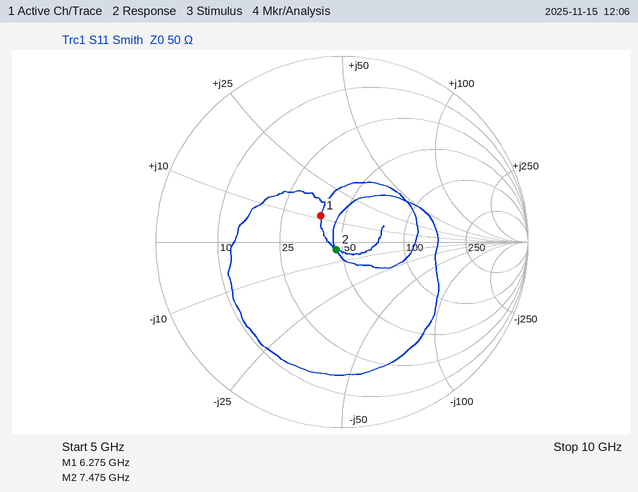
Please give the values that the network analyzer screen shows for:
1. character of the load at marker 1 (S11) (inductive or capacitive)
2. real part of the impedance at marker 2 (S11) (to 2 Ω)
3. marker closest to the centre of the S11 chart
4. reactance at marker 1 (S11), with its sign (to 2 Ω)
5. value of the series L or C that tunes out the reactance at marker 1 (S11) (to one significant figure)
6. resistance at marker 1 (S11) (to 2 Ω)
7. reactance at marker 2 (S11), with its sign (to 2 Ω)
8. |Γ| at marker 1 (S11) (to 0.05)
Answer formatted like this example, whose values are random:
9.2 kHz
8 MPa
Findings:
inductive
46 Ω
marker 2
+12 Ω
2 pF
38 Ω
-4 Ω
0.20
